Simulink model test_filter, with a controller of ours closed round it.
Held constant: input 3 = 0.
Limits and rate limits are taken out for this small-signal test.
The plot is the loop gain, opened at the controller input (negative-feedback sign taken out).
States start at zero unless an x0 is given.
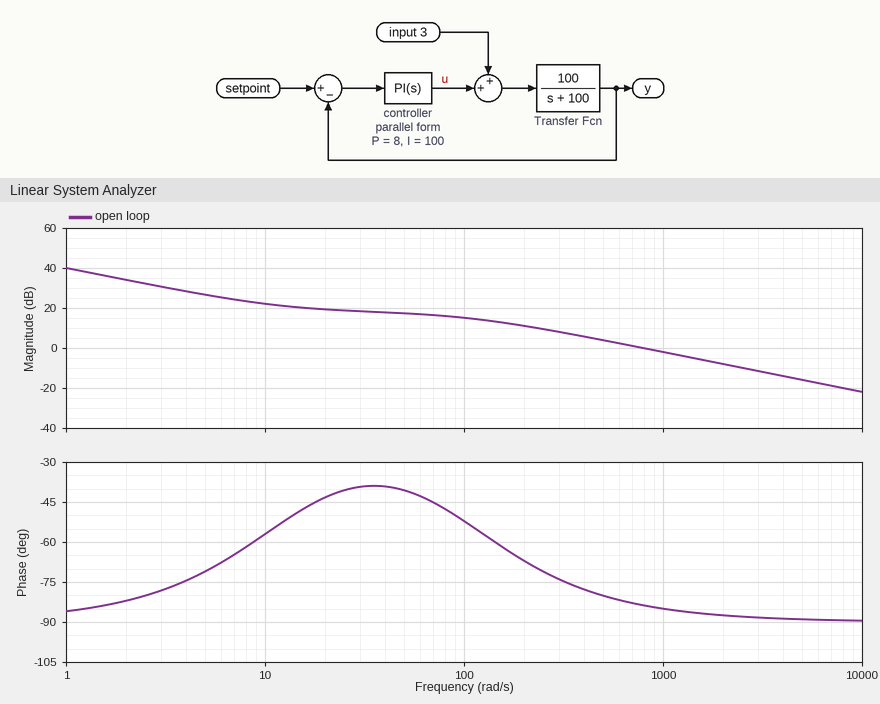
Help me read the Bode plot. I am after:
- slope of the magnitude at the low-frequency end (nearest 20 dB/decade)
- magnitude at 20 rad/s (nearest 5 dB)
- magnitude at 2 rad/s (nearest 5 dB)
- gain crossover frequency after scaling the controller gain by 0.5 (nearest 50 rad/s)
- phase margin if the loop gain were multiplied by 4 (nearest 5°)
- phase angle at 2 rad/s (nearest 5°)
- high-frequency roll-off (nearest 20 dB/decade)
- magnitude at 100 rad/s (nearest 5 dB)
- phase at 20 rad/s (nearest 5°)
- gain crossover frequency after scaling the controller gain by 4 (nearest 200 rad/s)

-20 dB/decade
20 dB
35 dB
400 rad/s
90°
-80°
-20 dB/decade
15 dB
-45°
3200 rad/s
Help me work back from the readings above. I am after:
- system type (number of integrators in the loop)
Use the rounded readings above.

1
